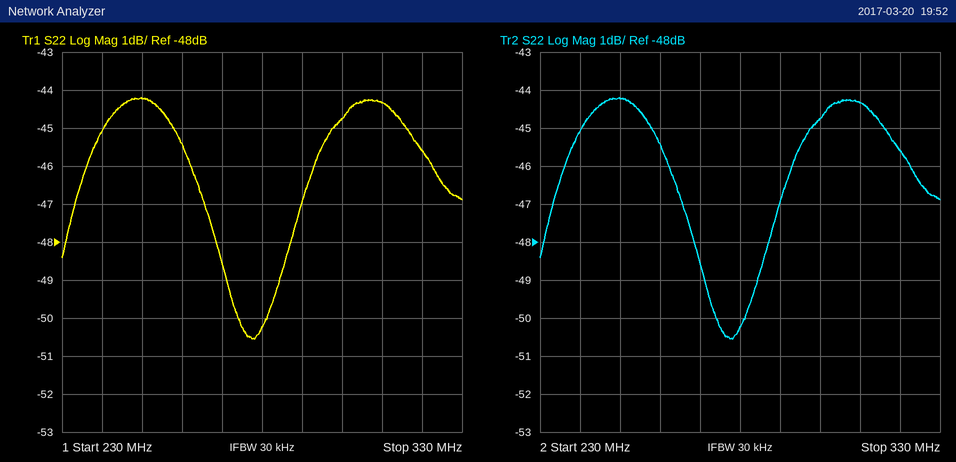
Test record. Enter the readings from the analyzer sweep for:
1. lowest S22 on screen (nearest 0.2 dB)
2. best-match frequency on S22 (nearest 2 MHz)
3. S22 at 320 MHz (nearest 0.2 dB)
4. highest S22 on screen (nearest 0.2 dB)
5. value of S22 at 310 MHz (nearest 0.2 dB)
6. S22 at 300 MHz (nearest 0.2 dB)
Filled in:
-50.6 dB
278 MHz
-45.6 dB
-44.2 dB
-44.4 dB
-44.8 dB
